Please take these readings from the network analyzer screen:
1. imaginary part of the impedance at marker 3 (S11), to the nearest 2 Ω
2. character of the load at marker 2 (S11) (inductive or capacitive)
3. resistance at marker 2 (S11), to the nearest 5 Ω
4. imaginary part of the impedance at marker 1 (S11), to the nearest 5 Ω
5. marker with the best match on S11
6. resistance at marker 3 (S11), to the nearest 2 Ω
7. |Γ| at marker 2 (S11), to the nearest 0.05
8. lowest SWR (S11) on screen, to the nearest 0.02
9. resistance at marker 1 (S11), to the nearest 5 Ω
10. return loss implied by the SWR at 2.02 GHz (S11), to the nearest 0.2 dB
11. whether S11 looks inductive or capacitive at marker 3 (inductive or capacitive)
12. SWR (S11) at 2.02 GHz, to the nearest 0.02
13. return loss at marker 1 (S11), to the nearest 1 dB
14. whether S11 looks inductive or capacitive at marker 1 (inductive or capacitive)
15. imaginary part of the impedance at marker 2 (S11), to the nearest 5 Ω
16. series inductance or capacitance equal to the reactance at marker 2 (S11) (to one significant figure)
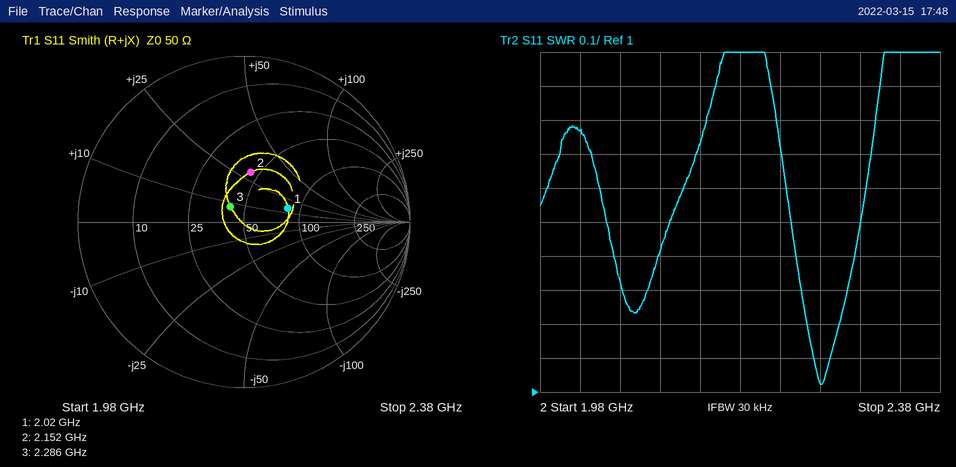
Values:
+8 Ω
inductive
45 Ω
+15 Ω
marker 3
42 Ω
0.30
1.02
85 Ω
11.2 dB
inductive
1.76
11 dB
inductive
+30 Ω
2 nH
